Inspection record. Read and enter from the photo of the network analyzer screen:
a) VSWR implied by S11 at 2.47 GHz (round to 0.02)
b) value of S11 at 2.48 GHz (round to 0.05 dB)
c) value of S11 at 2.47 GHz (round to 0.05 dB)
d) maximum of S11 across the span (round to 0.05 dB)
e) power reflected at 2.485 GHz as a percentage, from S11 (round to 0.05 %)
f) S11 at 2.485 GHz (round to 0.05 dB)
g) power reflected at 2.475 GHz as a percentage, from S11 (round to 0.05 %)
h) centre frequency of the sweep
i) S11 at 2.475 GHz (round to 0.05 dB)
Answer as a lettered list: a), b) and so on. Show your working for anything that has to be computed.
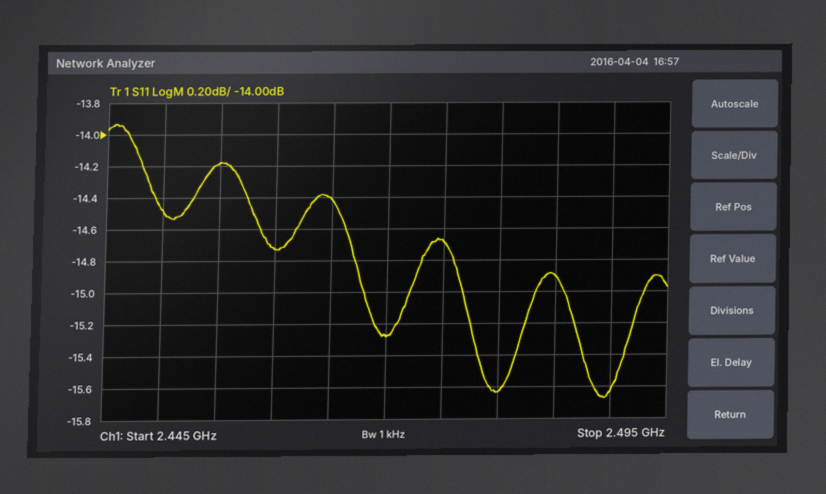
a) |Γ| = 10^(-15.3/20) = 0.1718; VSWR = (1 + 0.1718)/(1 − 0.1718) ≈ 1.41, so 1.42 to the nearest 0.02
b) -15.65 dB
c) -15.30 dB
d) -13.95 dB
e) 10^(-14.9/10) ≈ 3.24 %, so 3.25 % to the nearest 0.05 %
f) -14.90 dB
g) 10^(-14.7/10) ≈ 3.39 %, so 3.40 % to the nearest 0.05 %
h) 2.47 GHz
i) -14.70 dB
